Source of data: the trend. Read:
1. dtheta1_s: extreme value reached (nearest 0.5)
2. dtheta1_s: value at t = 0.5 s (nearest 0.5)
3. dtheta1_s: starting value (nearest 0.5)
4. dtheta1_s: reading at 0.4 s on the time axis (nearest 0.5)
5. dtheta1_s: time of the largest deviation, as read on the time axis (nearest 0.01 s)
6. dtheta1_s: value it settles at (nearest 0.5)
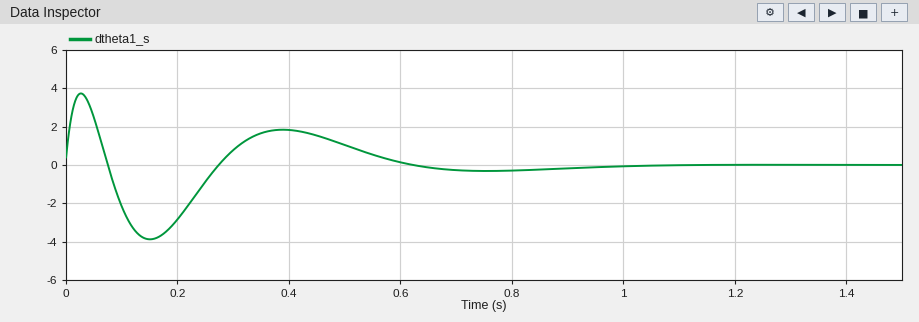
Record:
-4.0
1.0
0.5
2.0
0.15 s
0.0
